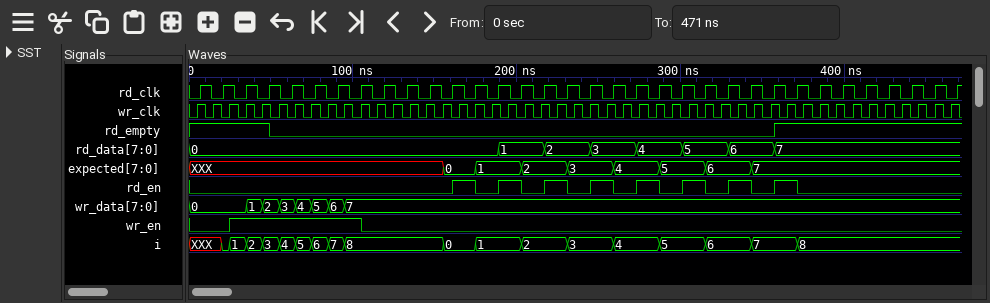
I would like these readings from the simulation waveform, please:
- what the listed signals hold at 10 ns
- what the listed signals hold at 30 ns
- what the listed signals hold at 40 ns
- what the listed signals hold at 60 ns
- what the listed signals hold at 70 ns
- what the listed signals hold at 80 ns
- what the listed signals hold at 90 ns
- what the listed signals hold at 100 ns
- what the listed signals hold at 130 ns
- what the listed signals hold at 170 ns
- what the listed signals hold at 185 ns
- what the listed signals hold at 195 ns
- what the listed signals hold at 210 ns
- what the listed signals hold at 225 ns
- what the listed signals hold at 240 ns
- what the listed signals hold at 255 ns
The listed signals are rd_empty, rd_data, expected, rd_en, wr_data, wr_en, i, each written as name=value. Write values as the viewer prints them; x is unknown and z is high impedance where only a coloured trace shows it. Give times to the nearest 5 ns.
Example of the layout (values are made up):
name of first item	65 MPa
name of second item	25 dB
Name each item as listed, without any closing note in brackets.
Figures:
what the listed signals hold at 10 ns	rd_empty=1, rd_data=0, expected=XXX, rd_en=0, wr_data=0, wr_en=0, i=XXX
what the listed signals hold at 30 ns	rd_empty=1, rd_data=0, expected=XXX, rd_en=0, wr_data=0, wr_en=1, i=1
what the listed signals hold at 40 ns	rd_empty=1, rd_data=0, expected=XXX, rd_en=0, wr_data=1, wr_en=1, i=2
what the listed signals hold at 60 ns	rd_empty=0, rd_data=0, expected=XXX, rd_en=0, wr_data=3, wr_en=1, i=4
what the listed signals hold at 70 ns	rd_empty=0, rd_data=0, expected=XXX, rd_en=0, wr_data=4, wr_en=1, i=5
what the listed signals hold at 80 ns	rd_empty=0, rd_data=0, expected=XXX, rd_en=0, wr_data=5, wr_en=1, i=6
what the listed signals hold at 90 ns	rd_empty=0, rd_data=0, expected=XXX, rd_en=0, wr_data=6, wr_en=1, i=7
what the listed signals hold at 100 ns	rd_empty=0, rd_data=0, expected=XXX, rd_en=0, wr_data=7, wr_en=1, i=8
what the listed signals hold at 130 ns	rd_empty=0, rd_data=0, expected=XXX, rd_en=0, wr_data=7, wr_en=0, i=8
what the listed signals hold at 170 ns	rd_empty=0, rd_data=0, expected=0, rd_en=1, wr_data=7, wr_en=0, i=0
what the listed signals hold at 185 ns	rd_empty=0, rd_data=0, expected=1, rd_en=0, wr_data=7, wr_en=0, i=1
what the listed signals hold at 195 ns	rd_empty=0, rd_data=1, expected=1, rd_en=1, wr_data=7, wr_en=0, i=1
what the listed signals hold at 210 ns	rd_empty=0, rd_data=1, expected=2, rd_en=0, wr_data=7, wr_en=0, i=2
what the listed signals hold at 225 ns	rd_empty=0, rd_data=2, expected=2, rd_en=1, wr_data=7, wr_en=0, i=2
what the listed signals hold at 240 ns	rd_empty=0, rd_data=2, expected=3, rd_en=0, wr_data=7, wr_en=0, i=3
what the listed signals hold at 255 ns	rd_empty=0, rd_data=3, expected=3, rd_en=1, wr_data=7, wr_en=0, i=3
